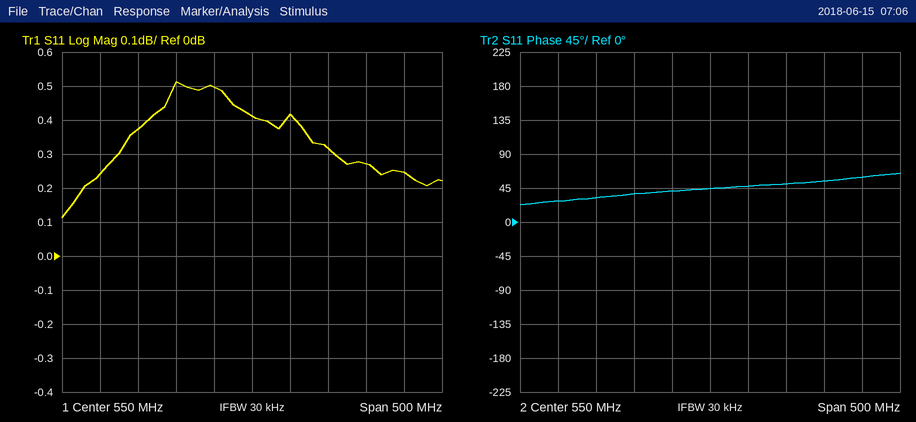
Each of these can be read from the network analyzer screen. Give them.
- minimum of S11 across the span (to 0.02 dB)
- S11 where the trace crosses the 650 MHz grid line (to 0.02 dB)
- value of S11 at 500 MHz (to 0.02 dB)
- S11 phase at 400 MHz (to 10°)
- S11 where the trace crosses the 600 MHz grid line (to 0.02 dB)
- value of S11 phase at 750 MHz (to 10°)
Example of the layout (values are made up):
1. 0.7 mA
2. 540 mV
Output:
1. 0.12 dB
2. 0.32 dB
3. 0.50 dB
4. 30°
5. 0.42 dB
6. 60°
